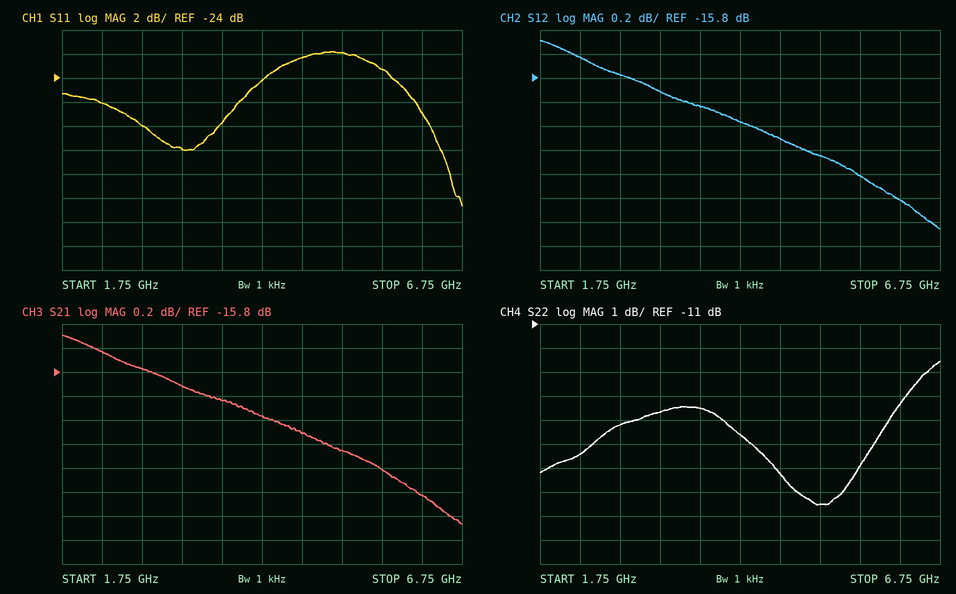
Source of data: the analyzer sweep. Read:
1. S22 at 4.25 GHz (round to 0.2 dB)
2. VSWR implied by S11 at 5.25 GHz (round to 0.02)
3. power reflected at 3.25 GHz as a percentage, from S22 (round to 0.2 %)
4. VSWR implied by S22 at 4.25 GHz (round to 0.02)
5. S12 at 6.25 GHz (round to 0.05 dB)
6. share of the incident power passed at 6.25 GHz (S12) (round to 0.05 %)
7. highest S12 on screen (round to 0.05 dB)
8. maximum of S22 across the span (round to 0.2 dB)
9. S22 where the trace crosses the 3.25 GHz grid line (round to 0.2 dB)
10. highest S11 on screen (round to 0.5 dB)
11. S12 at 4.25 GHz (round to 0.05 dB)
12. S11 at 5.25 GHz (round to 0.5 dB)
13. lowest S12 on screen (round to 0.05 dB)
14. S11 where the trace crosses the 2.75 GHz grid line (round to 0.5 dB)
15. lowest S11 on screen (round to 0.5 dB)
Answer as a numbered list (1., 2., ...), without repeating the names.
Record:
1. -15.6 dB
2. 1.18
3. 3.4 %
4. 1.40
5. -16.80 dB
6. 2.10 %
7. -15.50 dB
8. -12.6 dB
9. -14.6 dB
10. -22.0 dB
11. -16.15 dB
12. -22.0 dB
13. -17.05 dB
14. -28.0 dB
15. -34.5 dB
